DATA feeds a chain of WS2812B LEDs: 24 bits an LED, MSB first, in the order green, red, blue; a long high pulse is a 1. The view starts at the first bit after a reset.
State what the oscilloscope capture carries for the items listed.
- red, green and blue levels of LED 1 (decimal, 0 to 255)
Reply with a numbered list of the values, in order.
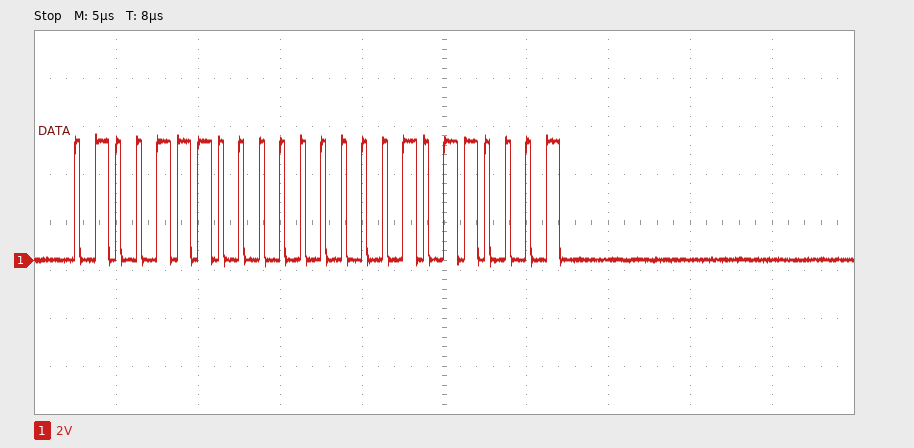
1. 0, 78, 177
